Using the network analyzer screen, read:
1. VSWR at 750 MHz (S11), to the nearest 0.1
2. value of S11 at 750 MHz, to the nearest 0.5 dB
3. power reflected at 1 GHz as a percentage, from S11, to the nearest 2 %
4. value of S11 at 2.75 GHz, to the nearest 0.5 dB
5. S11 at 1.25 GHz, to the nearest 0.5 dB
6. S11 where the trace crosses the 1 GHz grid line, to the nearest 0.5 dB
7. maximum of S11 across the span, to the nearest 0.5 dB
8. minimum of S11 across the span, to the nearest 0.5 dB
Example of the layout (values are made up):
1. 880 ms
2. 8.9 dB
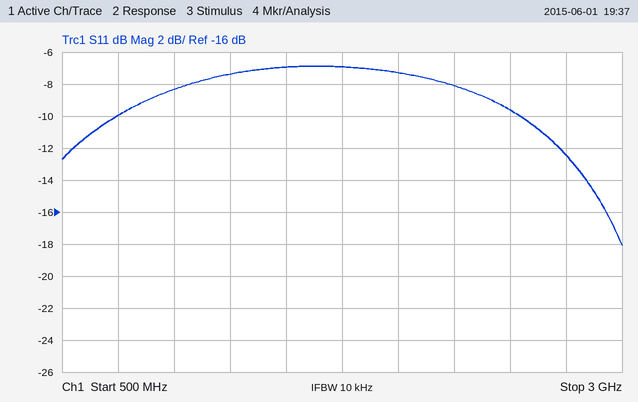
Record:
1. 1.9
2. -10.0 dB
3. 14 %
4. -12.5 dB
5. -7.5 dB
6. -8.5 dB
7. -7.0 dB
8. -18.0 dB
